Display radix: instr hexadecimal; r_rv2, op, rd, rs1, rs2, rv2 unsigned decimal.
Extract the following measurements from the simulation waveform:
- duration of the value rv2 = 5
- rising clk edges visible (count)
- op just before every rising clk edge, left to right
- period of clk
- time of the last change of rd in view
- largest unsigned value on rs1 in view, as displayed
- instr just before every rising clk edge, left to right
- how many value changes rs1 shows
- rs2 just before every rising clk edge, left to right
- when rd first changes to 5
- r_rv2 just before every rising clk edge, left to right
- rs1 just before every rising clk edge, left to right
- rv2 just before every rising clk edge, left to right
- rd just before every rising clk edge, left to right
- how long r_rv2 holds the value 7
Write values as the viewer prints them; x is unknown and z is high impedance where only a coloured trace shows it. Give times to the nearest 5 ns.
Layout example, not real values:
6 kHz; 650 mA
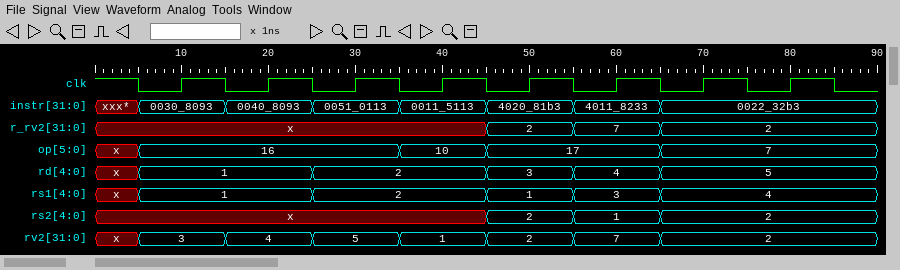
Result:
10 ns; 8; 16, 16, 16, 10, 17, 17, 7, 7; 10 ns; 65 ns; 4; 0030_8093, 0040_8093, 0051_0113, 0011_5113, 4020_81b3, 4011_8233, 0022_32b3, 0022_32b3; 5; x, x, x, x, 2, 1, 2, 2; 65 ns; x, x, x, x, 2, 7, 2, 2; 1, 1, 2, 2, 1, 3, 4, 4; 3, 4, 5, 1, 2, 7, 2, 2; 1, 1, 2, 2, 3, 4, 5, 5; 10 ns
